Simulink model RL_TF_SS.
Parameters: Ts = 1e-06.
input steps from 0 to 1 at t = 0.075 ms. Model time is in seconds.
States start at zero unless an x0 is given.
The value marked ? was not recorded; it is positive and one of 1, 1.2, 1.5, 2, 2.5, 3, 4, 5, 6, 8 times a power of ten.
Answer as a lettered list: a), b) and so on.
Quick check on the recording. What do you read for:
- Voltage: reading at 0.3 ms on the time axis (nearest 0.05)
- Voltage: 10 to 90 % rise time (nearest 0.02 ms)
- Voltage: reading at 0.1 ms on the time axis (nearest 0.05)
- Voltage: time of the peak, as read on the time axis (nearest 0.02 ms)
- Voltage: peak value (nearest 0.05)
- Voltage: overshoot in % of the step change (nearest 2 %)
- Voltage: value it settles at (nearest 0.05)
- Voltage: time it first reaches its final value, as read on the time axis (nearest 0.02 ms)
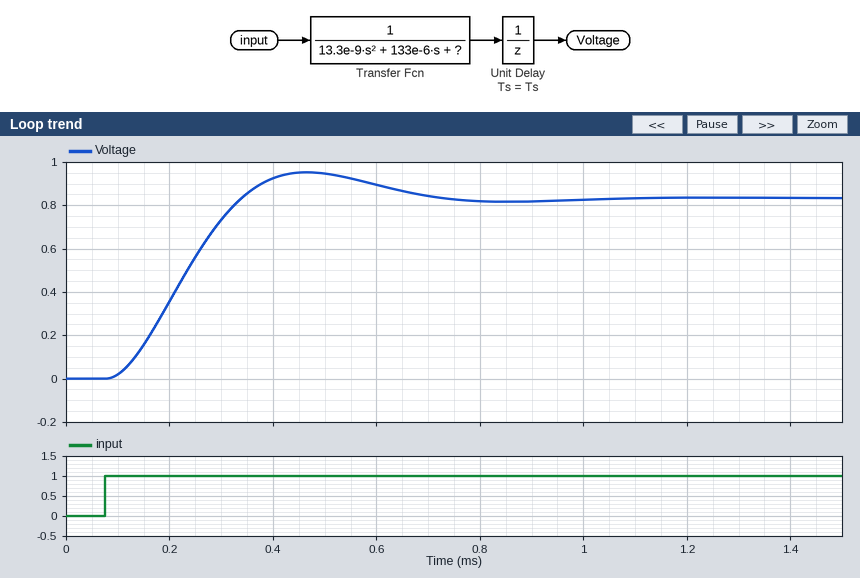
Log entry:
a) 0.75
b) 0.18 ms
c) 0.00
d) 0.46 ms
e) 0.95
f) 14 %
g) 0.85
h) 0.34 ms
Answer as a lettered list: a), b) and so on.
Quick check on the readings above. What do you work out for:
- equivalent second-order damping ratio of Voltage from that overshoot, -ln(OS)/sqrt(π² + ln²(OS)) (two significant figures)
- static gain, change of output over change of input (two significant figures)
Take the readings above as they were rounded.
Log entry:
a) 0.53
b) 0.85
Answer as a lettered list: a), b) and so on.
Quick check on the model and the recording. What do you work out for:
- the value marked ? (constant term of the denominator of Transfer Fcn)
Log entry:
a) 1.2
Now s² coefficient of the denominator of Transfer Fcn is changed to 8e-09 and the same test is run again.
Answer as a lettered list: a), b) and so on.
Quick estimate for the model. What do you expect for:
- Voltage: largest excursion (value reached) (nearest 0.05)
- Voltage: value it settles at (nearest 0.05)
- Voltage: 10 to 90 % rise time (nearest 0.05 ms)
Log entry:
a) 0.90
b) 0.85
c) 0.15 ms
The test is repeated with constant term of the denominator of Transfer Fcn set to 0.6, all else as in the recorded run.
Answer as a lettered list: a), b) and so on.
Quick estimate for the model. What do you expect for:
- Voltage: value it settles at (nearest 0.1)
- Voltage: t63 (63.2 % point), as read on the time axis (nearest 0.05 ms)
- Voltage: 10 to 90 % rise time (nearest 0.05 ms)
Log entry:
a) 1.7
b) 0.35 ms
c) 0.35 ms
